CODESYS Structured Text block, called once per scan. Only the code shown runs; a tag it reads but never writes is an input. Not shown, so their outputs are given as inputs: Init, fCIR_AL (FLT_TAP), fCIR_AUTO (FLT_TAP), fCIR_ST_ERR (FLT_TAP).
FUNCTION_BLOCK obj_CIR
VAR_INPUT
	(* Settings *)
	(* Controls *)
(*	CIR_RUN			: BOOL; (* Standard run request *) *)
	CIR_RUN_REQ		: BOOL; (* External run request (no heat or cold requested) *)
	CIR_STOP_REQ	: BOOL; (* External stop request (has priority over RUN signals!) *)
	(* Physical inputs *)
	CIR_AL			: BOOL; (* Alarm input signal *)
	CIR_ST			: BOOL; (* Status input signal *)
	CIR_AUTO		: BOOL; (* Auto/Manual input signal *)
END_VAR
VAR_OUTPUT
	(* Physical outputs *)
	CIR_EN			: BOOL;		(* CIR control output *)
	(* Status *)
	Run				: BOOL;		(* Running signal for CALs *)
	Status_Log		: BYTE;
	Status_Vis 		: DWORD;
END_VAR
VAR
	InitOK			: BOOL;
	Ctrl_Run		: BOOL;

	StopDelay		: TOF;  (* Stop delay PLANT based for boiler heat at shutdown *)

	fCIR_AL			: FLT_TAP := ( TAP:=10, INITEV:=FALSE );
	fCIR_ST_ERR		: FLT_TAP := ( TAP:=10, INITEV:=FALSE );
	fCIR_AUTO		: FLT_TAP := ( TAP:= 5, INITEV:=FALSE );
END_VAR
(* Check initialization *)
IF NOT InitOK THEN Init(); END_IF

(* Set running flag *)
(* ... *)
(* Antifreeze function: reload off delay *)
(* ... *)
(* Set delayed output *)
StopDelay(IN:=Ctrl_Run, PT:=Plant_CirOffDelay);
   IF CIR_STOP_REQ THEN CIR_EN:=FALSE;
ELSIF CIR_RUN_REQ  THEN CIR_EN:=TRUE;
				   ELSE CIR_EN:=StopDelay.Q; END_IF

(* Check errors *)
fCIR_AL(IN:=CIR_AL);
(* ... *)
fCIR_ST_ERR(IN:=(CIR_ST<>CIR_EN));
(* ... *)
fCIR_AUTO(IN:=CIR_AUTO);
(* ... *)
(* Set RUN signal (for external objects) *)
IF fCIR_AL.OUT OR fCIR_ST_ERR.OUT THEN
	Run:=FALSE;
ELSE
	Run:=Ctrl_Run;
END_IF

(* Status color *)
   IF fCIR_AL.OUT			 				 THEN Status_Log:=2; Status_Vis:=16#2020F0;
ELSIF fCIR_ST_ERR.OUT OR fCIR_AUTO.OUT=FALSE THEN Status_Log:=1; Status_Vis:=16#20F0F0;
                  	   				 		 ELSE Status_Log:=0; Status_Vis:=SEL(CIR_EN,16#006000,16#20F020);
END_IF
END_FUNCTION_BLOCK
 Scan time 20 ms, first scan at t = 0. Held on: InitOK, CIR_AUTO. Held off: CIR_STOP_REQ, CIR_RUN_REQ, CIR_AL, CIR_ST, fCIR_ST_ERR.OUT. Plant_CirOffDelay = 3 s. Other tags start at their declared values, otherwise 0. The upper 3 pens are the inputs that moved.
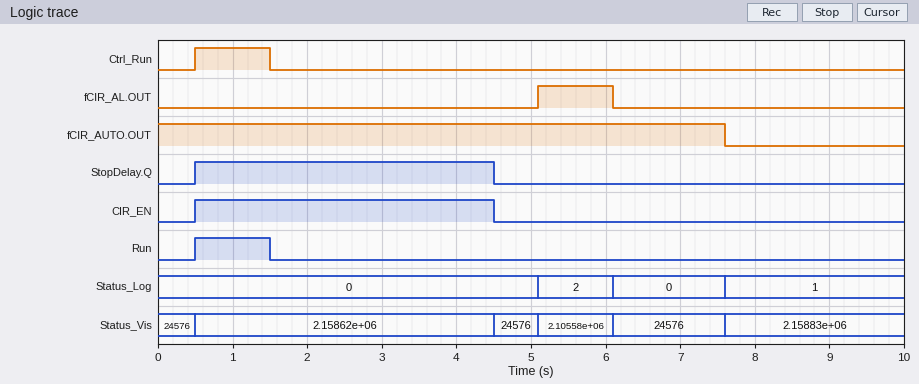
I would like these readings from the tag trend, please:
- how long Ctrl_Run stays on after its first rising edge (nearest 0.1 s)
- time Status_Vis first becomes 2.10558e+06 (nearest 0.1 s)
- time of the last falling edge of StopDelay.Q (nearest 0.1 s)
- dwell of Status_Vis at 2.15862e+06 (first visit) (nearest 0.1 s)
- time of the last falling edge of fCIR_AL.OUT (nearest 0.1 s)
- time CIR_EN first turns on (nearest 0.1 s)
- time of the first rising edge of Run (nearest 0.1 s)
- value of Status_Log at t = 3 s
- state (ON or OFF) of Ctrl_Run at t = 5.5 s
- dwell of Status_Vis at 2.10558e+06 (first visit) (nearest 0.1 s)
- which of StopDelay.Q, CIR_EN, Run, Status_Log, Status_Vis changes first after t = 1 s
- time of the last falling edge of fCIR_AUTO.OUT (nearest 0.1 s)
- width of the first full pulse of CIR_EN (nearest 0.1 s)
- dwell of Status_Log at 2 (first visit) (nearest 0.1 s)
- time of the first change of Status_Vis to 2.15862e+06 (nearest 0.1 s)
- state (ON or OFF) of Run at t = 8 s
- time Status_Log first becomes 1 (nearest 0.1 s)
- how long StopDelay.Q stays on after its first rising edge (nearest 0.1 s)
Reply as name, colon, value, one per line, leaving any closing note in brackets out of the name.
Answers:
how long Ctrl_Run stays on after its first rising edge: 1.0 s
time Status_Vis first becomes 2.10558e+06: 5.1 s
time of the last falling edge of StopDelay.Q: 4.5 s
dwell of Status_Vis at 2.15862e+06 (first visit): 4.0 s
time of the last falling edge of fCIR_AL.OUT: 6.1 s
time CIR_EN first turns on: 0.5 s
time of the first rising edge of Run: 0.5 s
value of Status_Log at t = 3 s: 0
state (ON or OFF) of Ctrl_Run at t = 5.5 s: OFF
dwell of Status_Vis at 2.10558e+06 (first visit): 1.0 s
which of StopDelay.Q, CIR_EN, Run, Status_Log, Status_Vis changes first after t = 1 s: Run
time of the last falling edge of fCIR_AUTO.OUT: 7.6 s
width of the first full pulse of CIR_EN: 4.0 s
dwell of Status_Log at 2 (first visit): 1.0 s
time of the first change of Status_Vis to 2.15862e+06: 0.5 s
state (ON or OFF) of Run at t = 8 s: OFF
time Status_Log first becomes 1: 7.6 s
how long StopDelay.Q stays on after its first rising edge: 4.0 s
